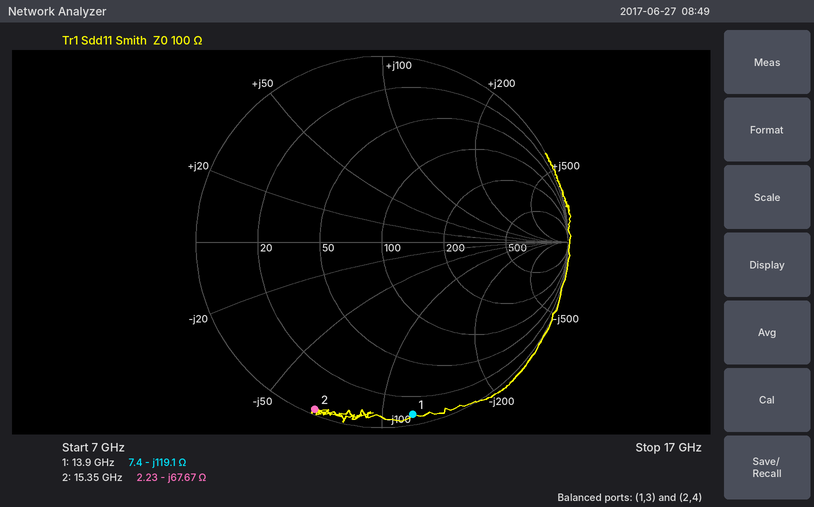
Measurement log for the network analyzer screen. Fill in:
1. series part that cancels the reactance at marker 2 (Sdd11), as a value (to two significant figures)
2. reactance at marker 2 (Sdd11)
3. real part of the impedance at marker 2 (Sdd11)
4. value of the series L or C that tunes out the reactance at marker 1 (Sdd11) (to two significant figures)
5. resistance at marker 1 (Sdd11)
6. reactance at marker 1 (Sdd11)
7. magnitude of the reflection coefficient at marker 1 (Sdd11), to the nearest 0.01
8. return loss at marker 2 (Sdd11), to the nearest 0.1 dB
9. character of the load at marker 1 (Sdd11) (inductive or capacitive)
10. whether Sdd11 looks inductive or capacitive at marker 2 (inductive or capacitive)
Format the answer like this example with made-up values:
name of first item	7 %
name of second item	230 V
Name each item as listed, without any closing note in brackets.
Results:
series part that cancels the reactance at marker 2 (Sdd11), as a value	700 pH
reactance at marker 2	-67.67 Ω
real part of the impedance at marker 2	2.23 Ω
value of the series L or C that tunes out the reactance at marker 1 (Sdd11)	1.4 nH
resistance at marker 1	7.4 Ω
reactance at marker 1	-119.1 Ω
magnitude of the reflection coefficient at marker 1 (Sdd11), to the nearest 0.01	0.94
return loss at marker 2 (Sdd11), to the nearest 0.1 dB	0.3 dB
character of the load at marker 1 (Sdd11)	capacitive
whether Sdd11 looks inductive or capacitive at marker 2	capacitive
